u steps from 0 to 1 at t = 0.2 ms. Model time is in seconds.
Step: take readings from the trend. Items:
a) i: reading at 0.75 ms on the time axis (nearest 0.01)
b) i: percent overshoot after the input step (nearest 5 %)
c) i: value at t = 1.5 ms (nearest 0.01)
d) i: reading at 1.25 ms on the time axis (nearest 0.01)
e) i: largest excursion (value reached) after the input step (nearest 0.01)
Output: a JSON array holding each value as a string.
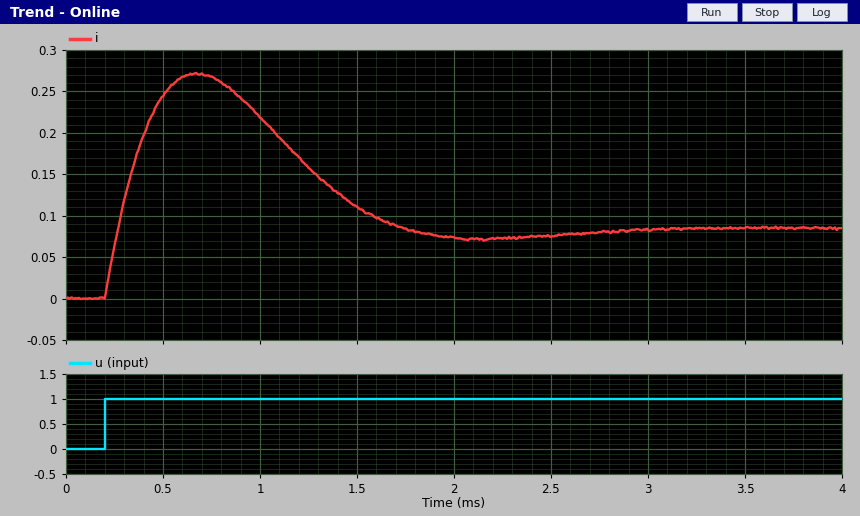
["0.27", "220 %", "0.11", "0.16", "0.27"]
